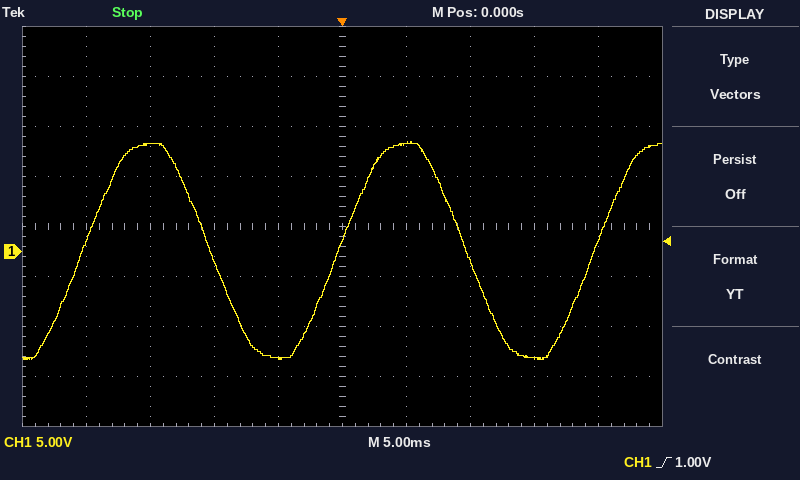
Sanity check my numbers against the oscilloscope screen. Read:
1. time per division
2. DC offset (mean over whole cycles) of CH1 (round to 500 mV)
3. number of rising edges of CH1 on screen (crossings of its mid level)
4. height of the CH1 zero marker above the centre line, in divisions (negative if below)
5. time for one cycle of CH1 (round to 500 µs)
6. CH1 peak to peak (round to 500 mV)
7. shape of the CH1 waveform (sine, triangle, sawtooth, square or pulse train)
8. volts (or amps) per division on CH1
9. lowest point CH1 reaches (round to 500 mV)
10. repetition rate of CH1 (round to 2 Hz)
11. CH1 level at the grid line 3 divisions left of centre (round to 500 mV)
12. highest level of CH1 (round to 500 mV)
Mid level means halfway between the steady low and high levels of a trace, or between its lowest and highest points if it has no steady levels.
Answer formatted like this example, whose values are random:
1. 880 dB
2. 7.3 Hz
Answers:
1. 5 ms
2. 0.0 V
3. 3
4. -0.5 div
5. 20.0 ms
6. 22.0 V
7. sine
8. 5 V
9. -11.0 V
10. 50 Hz
11. 11.0 V
12. 11.0 V
